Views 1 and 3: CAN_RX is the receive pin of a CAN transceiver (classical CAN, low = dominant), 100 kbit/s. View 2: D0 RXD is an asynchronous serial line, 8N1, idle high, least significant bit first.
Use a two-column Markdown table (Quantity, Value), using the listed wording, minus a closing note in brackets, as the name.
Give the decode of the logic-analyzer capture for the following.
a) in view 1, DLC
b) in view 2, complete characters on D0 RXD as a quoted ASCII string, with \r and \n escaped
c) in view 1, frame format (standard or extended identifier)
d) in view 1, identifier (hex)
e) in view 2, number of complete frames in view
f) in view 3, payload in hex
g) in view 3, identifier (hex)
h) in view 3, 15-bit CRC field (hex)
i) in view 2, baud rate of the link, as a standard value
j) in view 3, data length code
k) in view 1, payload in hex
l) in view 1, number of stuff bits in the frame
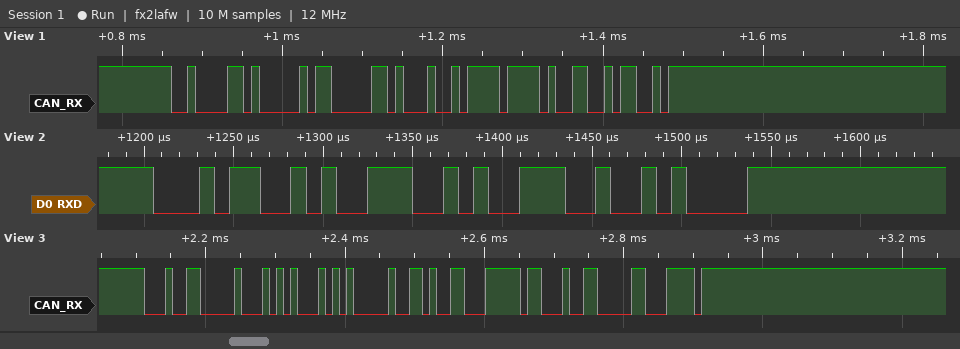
| Quantity | Value |
|---|---|
| in view 1, DLC | 3 |
| in view 2, complete characters on D0 RXD as a quoted ASCII string, with \r and \n escaped | "499\n" |
| in view 1, frame format | standard |
| in view 1, identifier | 0x21A |
| in view 2, number of complete frames in view | 4 |
| in view 3, payload in hex | 45 40 69 8F E2 |
| in view 3, identifier | 0x130 |
| in view 3, 15-bit CRC field | 0x3047 |
| in view 2, baud rate of the link, as a standard value | 115200 baud |
| in view 3, data length code | 5 |
| in view 1, payload in hex | 05 12 F7 |
| in view 1, number of stuff bits in the frame | 2 |
